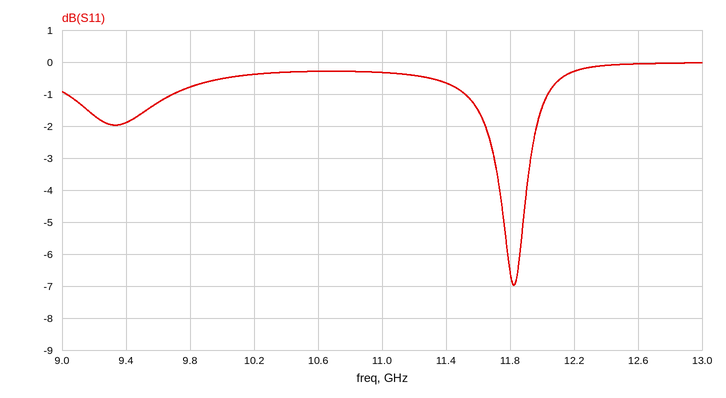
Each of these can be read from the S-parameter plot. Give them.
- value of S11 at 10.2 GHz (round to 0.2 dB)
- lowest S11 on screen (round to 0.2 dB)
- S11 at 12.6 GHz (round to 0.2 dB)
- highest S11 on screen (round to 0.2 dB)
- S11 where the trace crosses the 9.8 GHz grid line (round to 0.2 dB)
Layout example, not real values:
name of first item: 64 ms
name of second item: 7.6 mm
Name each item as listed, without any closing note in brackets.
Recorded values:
value of S11 at 10.2 GHz: -0.4 dB
lowest S11 on screen: -7.0 dB
S11 at 12.6 GHz: 0.0 dB
highest S11 on screen: 0.0 dB
S11 where the trace crosses the 9.8 GHz grid line: -0.8 dB
